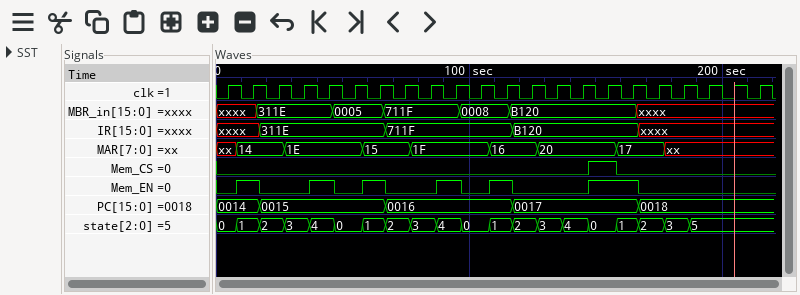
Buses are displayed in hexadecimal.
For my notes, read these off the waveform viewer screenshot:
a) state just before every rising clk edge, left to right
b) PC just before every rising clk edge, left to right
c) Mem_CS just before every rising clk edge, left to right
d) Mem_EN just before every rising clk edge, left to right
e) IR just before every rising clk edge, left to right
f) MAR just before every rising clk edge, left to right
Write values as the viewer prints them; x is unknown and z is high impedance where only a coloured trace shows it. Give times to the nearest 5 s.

0, 1, 2, 3, 4, 0, 1, 2, 3, 4, 0, 1, 2, 3, 4, 0, 1, 2, 3, 5, 5, 5
0014, 0014, 0015, 0015, 0015, 0015, 0015, 0016, 0016, 0016, 0016, 0016, 0017, 0017, 0017, 0017, 0017, 0018, 0018, 0018, 0018, 0018
0 0 0 0 0 0 0 0 0 0 0 0 0 0 0 1 0 0 0 0 0 0
0 1 0 0 1 0 1 0 0 1 0 1 0 0 0 1 1 0 0 0 0 0
xxxx, xxxx, 311E, 311E, 311E, 311E, 311E, 711F, 711F, 711F, 711F, 711F, B120, B120, B120, B120, B120, xxxx, xxxx, xxxx, xxxx, xxxx
xx, 14, 14, 1E, 1E, 1E, 15, 15, 1F, 1F, 1F, 16, 16, 20, 20, 20, 17, 17, xx, xx, xx, xx
